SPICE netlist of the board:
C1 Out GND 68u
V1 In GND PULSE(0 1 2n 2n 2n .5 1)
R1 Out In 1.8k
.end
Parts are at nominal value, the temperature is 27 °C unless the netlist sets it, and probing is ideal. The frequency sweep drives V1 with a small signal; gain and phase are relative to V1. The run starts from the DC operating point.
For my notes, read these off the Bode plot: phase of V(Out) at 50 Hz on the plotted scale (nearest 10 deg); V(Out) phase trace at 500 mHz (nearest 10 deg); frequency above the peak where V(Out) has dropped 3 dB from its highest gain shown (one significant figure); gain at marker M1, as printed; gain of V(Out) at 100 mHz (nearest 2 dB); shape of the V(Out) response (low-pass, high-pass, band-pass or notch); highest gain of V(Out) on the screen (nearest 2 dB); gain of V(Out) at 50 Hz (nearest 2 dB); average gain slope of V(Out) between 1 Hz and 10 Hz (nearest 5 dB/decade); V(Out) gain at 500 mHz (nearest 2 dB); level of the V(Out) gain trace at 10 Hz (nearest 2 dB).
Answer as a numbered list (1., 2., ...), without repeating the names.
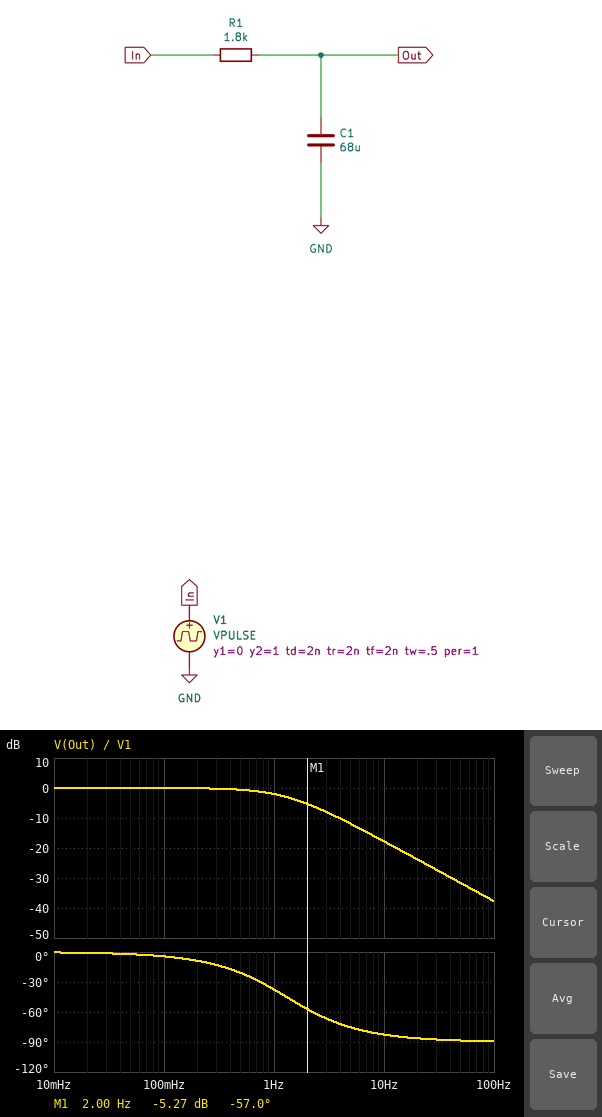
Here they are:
1. -90 deg
2. -20 deg
3. 1 Hz
4. -5.27 dB
5. 0 dB
6. low-pass
7. 0 dB
8. -32 dB
9. -15 dB/decade
10. 0 dB
11. -18 dB
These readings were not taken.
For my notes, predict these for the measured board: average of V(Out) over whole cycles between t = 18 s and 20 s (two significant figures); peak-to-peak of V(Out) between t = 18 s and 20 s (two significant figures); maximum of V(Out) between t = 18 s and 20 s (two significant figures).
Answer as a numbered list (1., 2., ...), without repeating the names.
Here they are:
1. 500 mV
2. 970 mV
3. 980 mV
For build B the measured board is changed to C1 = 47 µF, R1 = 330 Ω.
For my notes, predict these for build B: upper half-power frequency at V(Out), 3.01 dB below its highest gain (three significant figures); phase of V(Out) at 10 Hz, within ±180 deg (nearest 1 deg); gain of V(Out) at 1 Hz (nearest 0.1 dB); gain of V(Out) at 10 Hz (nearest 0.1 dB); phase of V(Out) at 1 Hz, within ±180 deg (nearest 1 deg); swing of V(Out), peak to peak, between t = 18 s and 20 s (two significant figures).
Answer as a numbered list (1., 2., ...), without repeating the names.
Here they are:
1. 10.3 Hz
2. -44 deg
3. 0 dB
4. -2.9 dB
5. -6 deg
6. 1.0 V
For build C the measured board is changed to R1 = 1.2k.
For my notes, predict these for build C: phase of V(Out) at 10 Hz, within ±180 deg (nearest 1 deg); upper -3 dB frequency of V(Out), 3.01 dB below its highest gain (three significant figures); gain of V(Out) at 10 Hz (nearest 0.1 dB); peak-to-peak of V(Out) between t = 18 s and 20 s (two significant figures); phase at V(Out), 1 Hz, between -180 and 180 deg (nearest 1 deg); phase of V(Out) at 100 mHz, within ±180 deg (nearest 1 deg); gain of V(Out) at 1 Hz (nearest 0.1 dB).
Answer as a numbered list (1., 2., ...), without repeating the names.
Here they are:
1. -79 deg
2. 1.95 Hz
3. -14.4 dB
4. 1.0 V
5. -27 deg
6. -3 deg
7. -1.0 dB
